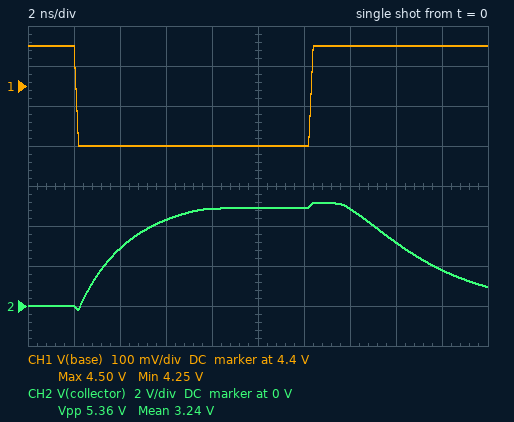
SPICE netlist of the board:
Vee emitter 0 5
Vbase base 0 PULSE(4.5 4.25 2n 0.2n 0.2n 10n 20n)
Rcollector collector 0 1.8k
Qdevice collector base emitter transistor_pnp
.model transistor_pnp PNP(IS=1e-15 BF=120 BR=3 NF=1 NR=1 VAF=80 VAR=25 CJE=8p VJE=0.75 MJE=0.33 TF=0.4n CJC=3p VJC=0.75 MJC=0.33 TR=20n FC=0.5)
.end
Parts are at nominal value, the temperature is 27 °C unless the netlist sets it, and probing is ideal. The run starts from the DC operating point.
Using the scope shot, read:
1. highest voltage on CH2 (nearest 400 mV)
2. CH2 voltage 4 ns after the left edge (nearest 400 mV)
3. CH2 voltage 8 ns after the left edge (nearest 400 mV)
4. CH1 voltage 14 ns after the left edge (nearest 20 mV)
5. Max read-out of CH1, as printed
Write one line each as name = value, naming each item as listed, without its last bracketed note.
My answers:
highest voltage on CH2 = 5.2 V
CH2 voltage 4 ns after the left edge = 2.8 V
CH2 voltage 8 ns after the left edge = 4.8 V
CH1 voltage 14 ns after the left edge = 4.50 V
Max read-out of CH1, as printed = 4.50 V
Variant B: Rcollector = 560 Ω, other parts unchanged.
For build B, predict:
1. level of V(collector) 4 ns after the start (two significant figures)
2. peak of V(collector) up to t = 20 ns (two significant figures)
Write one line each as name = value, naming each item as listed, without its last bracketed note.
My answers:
level of V(collector) 4 ns after the start = 1.8 V
peak of V(collector) up to t = 20 ns = 2.2 V
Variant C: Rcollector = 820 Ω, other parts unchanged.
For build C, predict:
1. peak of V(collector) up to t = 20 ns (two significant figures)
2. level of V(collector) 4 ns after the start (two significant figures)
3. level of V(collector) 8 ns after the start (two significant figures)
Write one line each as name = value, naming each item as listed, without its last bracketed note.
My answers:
peak of V(collector) up to t = 20 ns = 3.2 V
level of V(collector) 4 ns after the start = 2.2 V
level of V(collector) 8 ns after the start = 3.1 V
